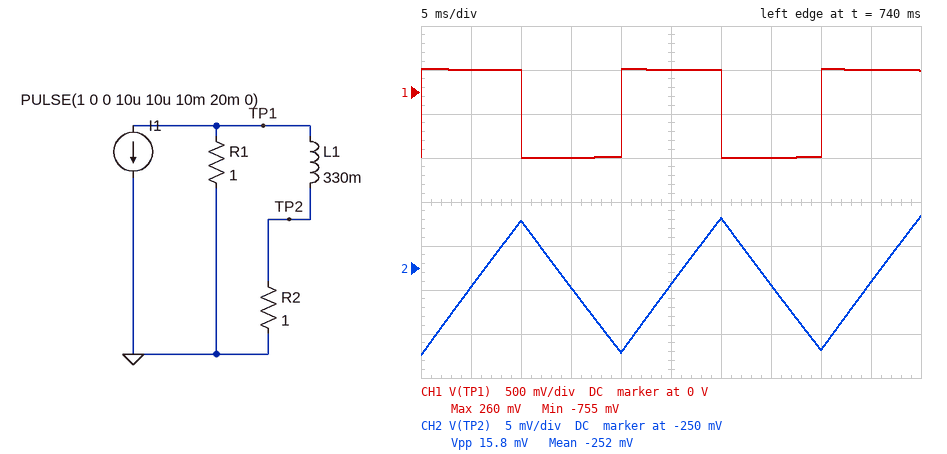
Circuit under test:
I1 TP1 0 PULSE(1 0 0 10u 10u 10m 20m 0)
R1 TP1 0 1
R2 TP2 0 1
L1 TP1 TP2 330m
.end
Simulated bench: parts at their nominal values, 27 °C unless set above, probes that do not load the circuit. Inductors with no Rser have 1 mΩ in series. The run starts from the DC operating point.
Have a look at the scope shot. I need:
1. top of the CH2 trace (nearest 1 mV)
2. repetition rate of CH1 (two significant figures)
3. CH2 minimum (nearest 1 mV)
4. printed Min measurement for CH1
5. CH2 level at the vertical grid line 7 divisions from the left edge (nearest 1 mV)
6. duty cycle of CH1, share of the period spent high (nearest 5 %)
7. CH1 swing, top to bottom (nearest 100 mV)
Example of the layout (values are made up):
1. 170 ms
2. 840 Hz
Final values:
1. -244 mV
2. 50 Hz
3. -260 mV
4. -755 mV
5. -252 mV
6. 50 %
7. 1.0 V
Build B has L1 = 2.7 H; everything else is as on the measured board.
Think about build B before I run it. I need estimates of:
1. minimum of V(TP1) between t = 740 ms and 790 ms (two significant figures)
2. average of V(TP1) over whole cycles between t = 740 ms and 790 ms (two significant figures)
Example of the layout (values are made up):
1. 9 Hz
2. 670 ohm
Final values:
1. -610 mV
2. -110 mV
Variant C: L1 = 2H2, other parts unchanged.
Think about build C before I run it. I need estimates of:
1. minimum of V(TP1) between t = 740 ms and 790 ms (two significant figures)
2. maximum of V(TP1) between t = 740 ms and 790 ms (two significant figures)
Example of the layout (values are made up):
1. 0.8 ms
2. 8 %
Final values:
1. -630 mV
2. 380 mV
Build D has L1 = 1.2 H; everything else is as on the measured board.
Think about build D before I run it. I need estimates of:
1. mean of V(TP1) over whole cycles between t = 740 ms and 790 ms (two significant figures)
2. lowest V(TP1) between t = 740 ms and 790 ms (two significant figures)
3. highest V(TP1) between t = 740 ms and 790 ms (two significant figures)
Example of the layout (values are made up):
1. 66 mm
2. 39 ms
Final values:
1. -180 mV
2. -680 mV
3. 320 mV
